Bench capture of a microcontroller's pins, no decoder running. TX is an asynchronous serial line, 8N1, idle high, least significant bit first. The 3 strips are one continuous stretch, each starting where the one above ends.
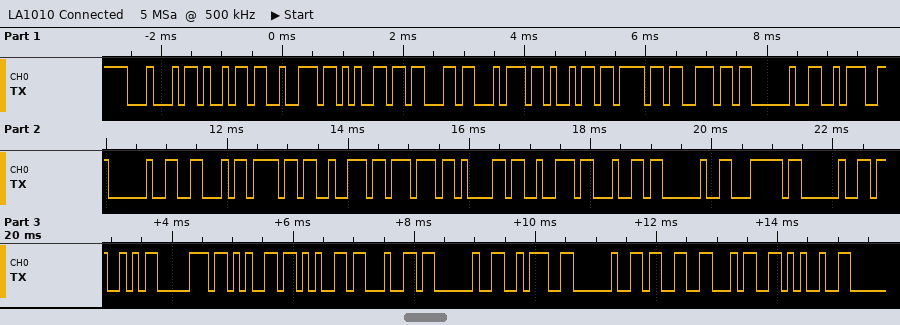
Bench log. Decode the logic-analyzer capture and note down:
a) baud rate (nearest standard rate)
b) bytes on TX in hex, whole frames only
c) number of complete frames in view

9600 baud
0x44 0x69 0x72 0x65 0x63 0x74 0x69 0x6F 0x6E 0x20 0x3A 0x20 0x46 0x6F 0x72 0x77 0x61 0x72 0x64 0x20 0x7C 0x20 0x53 0x70 0x65 0x65 0x64 0x20 0x3A 0x20 0x33 0x34 0x25
33
